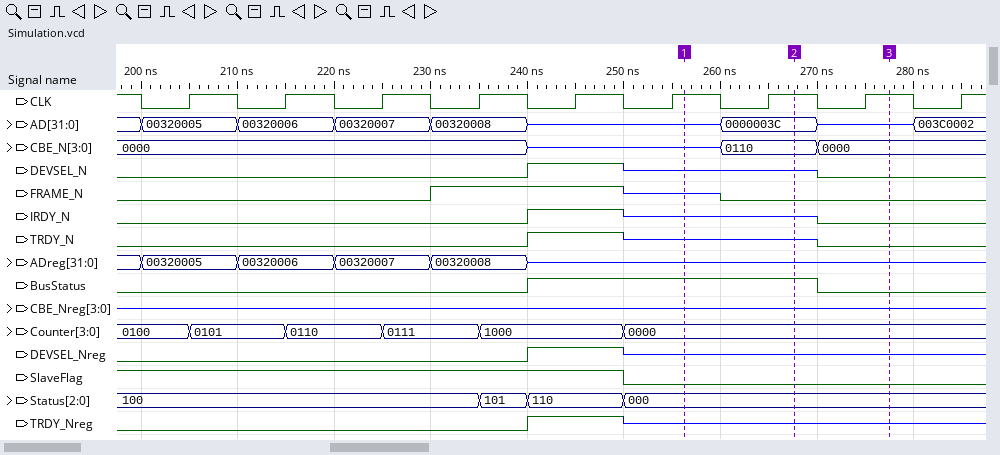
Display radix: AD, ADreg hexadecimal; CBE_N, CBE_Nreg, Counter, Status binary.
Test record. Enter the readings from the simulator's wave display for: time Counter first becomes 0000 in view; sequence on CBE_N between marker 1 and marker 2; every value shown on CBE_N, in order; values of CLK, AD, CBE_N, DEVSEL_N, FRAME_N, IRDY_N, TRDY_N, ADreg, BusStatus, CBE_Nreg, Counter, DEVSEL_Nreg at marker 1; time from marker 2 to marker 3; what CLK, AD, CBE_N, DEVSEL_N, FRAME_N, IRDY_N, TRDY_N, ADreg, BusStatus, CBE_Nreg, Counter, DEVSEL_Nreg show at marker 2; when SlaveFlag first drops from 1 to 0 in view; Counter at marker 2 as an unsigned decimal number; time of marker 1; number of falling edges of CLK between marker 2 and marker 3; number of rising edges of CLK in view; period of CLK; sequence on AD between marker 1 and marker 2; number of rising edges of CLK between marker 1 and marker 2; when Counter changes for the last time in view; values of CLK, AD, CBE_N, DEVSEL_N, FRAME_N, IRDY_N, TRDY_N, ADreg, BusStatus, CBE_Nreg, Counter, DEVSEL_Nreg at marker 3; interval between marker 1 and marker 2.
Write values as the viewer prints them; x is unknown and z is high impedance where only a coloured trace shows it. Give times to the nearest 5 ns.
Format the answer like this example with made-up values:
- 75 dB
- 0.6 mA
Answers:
- 250 ns
- z, 0110
- 0000, z, 0110, 0000
- CLK=1, AD=z, CBE_N=z, DEVSEL_N=z, FRAME_N=z, IRDY_N=z, TRDY_N=z, ADreg=z, BusStatus=1, CBE_Nreg=z, Counter=0000, DEVSEL_Nreg=z
- 10 ns
- CLK=1, AD=0000003C, CBE_N=0110, DEVSEL_N=z, FRAME_N=0, IRDY_N=z, TRDY_N=z, ADreg=z, BusStatus=1, CBE_Nreg=z, Counter=0000, DEVSEL_Nreg=z
- 250 ns
- 0
- 255 ns
- 1
- 9
- 10 ns
- z, 0000003C
- 1
- 250 ns
- CLK=1, AD=z, CBE_N=0000, DEVSEL_N=0, FRAME_N=0, IRDY_N=0, TRDY_N=0, ADreg=z, BusStatus=0, CBE_Nreg=z, Counter=0000, DEVSEL_Nreg=z
- 10 ns
